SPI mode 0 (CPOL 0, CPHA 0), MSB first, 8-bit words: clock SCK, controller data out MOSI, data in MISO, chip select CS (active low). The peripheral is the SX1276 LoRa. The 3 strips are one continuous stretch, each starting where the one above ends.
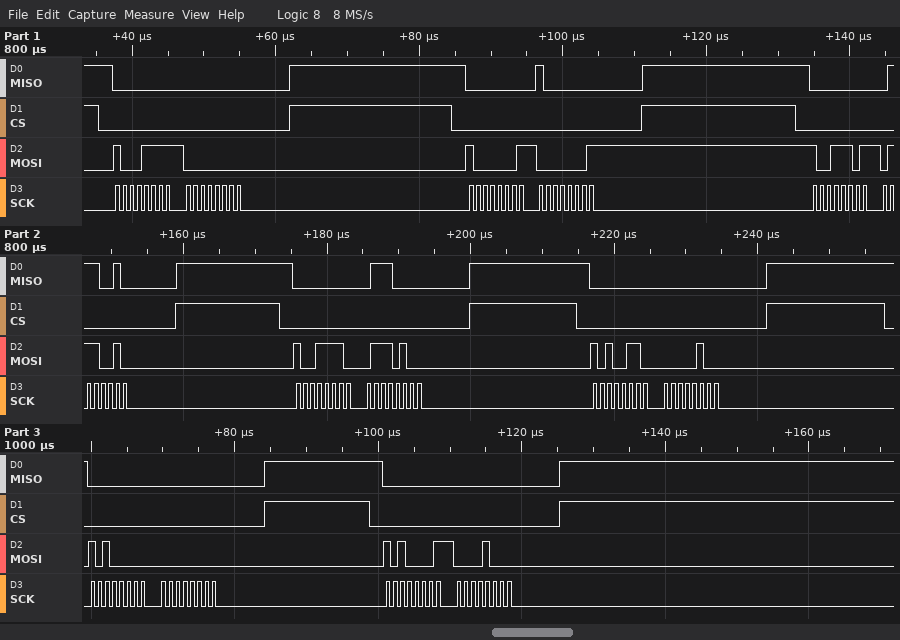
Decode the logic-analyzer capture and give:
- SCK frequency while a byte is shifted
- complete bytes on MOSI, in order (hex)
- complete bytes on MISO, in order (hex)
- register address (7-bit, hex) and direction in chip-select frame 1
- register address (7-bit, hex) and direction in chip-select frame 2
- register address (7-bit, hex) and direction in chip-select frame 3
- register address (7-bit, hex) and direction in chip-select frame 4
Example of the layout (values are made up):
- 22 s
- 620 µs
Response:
- 1 MHz
- 0x8F 0x00 0x81 0x01 0x9D 0x72 0x9E 0x74 0xA6 0x04 0xA0 0x00 0xA1 0x08
- 0x00 0x00 0x00 0x80 0x00 0x72 0x00 0x70 0x00 0x00 0x00 0x00 0x00 0x00
- 0x0F write
- 0x01 write
- 0x1D write
- 0x1E write
